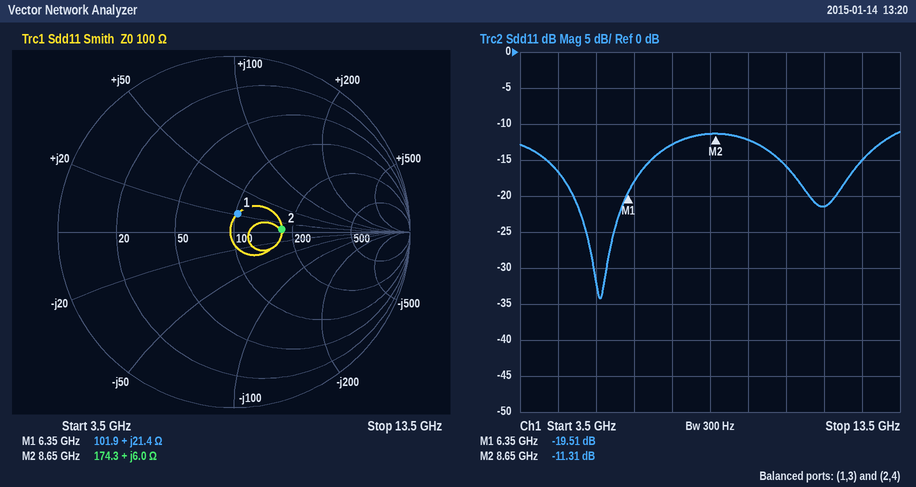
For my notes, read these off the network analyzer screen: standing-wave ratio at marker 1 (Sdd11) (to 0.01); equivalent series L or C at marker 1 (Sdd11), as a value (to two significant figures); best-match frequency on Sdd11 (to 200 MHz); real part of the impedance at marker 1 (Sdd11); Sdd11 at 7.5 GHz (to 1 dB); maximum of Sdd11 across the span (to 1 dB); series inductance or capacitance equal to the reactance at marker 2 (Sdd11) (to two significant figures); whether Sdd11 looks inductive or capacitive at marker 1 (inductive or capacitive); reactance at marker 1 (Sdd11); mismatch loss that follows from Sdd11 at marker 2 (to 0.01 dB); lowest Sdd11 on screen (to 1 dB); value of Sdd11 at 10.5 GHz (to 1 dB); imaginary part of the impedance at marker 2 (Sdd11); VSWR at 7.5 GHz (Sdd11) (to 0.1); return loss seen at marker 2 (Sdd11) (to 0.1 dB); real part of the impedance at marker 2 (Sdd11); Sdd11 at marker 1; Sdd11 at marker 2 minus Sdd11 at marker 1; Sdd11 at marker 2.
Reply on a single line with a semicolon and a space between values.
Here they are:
1.24; 540 pH; 5.6 GHz; 101.9 Ω; -13 dB; -11 dB; 110 pH; inductive; +21.4 Ω; 0.33 dB; -34 dB; -16 dB; +6.0 Ω; 1.6; 11.3 dB; 174.3 Ω; -19.51 dB; 8.20 dB; -11.31 dB
